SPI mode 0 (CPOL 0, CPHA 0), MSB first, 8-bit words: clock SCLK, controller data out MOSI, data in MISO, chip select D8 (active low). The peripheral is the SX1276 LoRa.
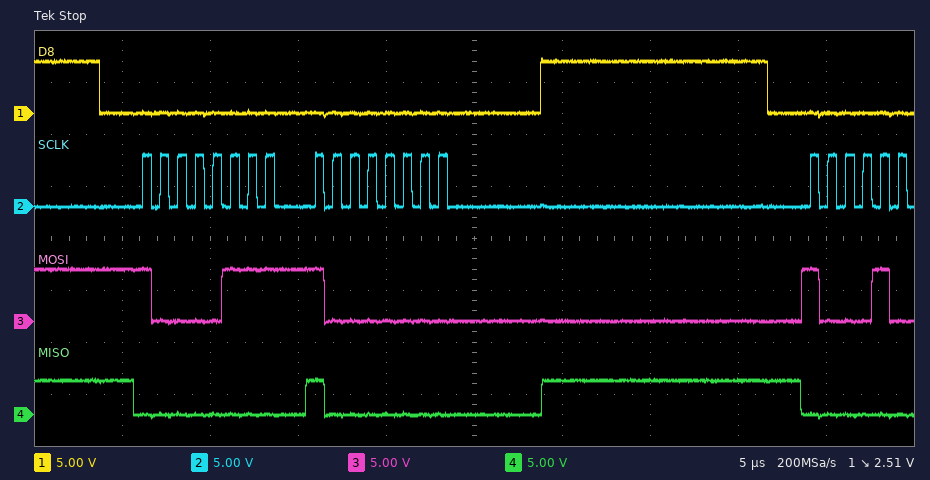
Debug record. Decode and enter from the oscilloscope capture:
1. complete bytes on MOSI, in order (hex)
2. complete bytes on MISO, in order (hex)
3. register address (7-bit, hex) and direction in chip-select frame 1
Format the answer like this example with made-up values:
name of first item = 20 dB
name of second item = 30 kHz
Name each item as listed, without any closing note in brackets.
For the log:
complete bytes on MOSI, in order = 0x87 0x80
complete bytes on MISO, in order = 0x00 0x80
register address (7-bit, hex) and direction in chip-select frame 1 = 0x07 write
